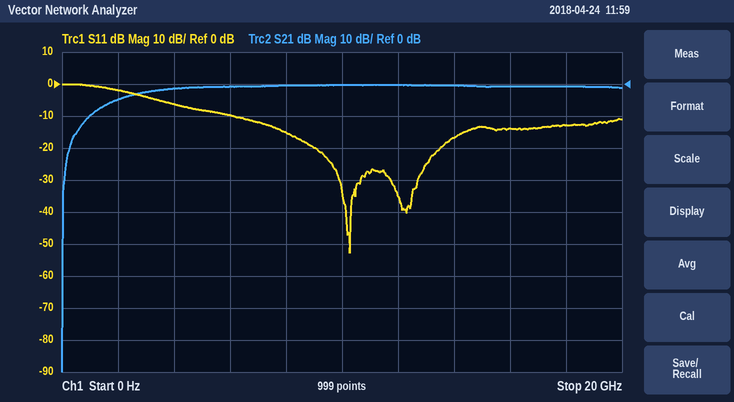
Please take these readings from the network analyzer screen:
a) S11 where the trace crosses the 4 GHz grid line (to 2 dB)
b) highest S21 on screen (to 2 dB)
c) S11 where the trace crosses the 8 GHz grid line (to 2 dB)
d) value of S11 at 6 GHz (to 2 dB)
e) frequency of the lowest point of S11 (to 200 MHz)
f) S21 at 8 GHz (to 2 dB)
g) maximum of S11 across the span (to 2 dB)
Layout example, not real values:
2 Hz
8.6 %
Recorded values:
-6 dB
0 dB
-16 dB
-10 dB
10.2 GHz
0 dB
0 dB
